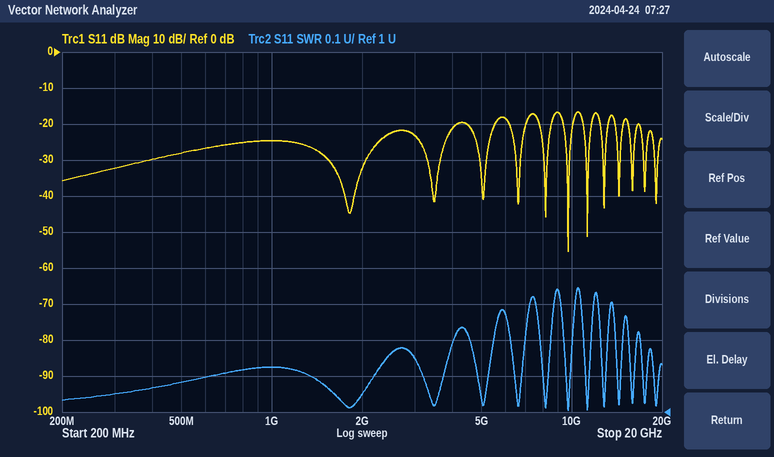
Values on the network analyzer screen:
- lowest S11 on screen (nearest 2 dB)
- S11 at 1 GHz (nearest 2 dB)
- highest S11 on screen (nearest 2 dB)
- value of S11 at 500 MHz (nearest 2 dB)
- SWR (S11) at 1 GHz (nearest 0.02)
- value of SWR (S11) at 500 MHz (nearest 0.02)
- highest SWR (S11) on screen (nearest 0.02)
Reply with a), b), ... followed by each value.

a) -56 dB
b) -24 dB
c) -16 dB
d) -28 dB
e) 1.12
f) 1.08
g) 1.34
